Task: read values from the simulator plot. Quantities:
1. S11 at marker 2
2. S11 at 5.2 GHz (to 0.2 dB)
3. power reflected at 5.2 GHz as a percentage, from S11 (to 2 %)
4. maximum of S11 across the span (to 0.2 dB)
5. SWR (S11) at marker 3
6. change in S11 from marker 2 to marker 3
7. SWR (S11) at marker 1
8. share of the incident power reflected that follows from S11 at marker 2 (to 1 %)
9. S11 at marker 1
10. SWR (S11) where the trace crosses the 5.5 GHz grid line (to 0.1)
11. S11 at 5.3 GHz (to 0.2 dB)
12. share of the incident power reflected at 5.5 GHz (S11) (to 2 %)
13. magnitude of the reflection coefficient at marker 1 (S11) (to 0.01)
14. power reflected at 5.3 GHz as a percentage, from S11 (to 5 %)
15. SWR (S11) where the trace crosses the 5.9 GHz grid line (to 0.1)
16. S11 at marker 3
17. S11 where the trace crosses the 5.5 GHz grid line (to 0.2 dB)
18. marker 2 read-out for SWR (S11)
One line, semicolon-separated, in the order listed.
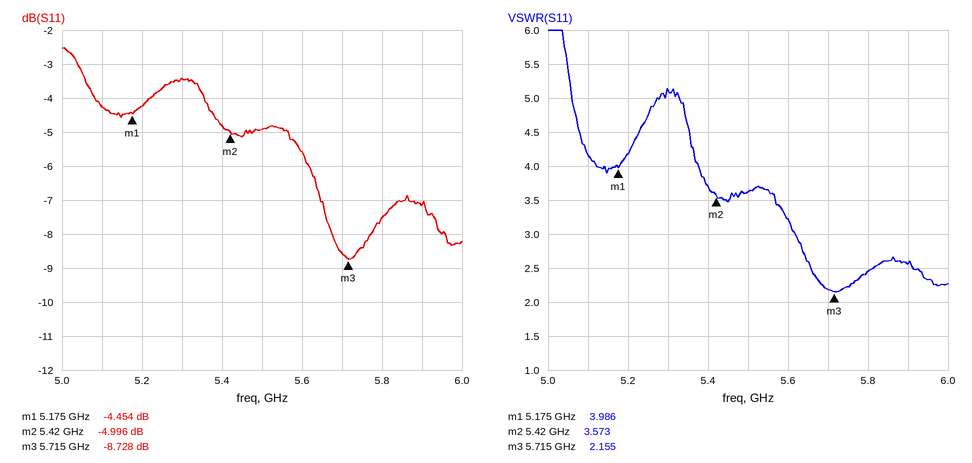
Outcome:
-4.996 dB; -4.2 dB; 38 %; -2.6 dB; 2.155; -3.732 dB; 3.986; 32 %; -4.454 dB; 3.6; -3.4 dB; 32 %; 0.60; 45 %; 2.6; -8.728 dB; -5.0 dB; 3.573
